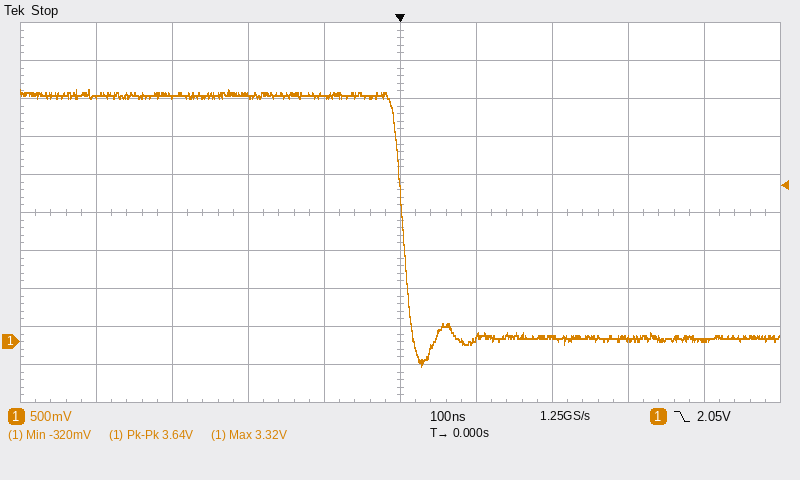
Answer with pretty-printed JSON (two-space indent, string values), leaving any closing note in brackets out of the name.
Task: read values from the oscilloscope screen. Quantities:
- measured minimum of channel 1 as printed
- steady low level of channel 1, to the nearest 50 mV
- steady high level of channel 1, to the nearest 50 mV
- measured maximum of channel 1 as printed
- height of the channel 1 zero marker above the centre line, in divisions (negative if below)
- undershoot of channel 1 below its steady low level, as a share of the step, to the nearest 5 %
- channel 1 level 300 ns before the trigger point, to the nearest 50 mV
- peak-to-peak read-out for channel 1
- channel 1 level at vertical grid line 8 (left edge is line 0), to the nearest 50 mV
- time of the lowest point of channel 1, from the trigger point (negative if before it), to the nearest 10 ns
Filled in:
{
  "measured minimum of channel 1 as printed": "-320 mV",
  "steady low level of channel 1, to the nearest 50 mV": "50 mV",
  "steady high level of channel 1, to the nearest 50 mV": "3.25 V",
  "measured maximum of channel 1 as printed": "3.32 V",
  "height of the channel 1 zero marker above the centre line, in divisions": "-3.4 div",
  "undershoot of channel 1 below its steady low level, as a share of the step, to the nearest 5 %": "10 %",
  "channel 1 level 300 ns before the trigger point, to the nearest 50 mV": "3.25 V",
  "peak-to-peak read-out for channel 1": "3.64 V",
  "channel 1 level at vertical grid line 8 (left edge is line 0), to the nearest 50 mV": "50 mV",
  "time of the lowest point of channel 1, from the trigger point (negative if before it), to the nearest 10 ns": "+30 ns"
}
